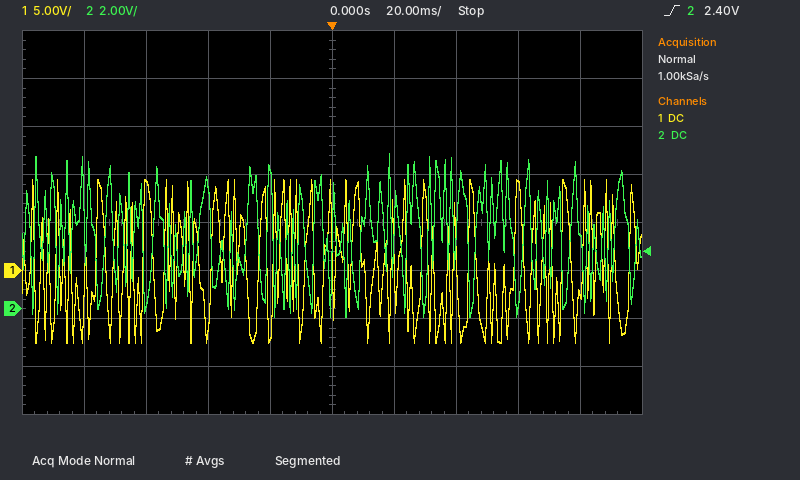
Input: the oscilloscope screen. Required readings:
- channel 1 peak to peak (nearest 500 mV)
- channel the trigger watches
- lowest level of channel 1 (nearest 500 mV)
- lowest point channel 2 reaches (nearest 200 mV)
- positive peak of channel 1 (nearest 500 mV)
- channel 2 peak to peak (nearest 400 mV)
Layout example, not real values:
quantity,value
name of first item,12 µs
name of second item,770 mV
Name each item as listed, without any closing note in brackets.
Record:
quantity,value
channel 1 peak to peak,17.0 V
channel the trigger watches,channel 2
lowest level of channel 1,-7.5 V
lowest point channel 2 reaches,-400 mV
positive peak of channel 1,9.5 V
channel 2 peak to peak,6.8 V
